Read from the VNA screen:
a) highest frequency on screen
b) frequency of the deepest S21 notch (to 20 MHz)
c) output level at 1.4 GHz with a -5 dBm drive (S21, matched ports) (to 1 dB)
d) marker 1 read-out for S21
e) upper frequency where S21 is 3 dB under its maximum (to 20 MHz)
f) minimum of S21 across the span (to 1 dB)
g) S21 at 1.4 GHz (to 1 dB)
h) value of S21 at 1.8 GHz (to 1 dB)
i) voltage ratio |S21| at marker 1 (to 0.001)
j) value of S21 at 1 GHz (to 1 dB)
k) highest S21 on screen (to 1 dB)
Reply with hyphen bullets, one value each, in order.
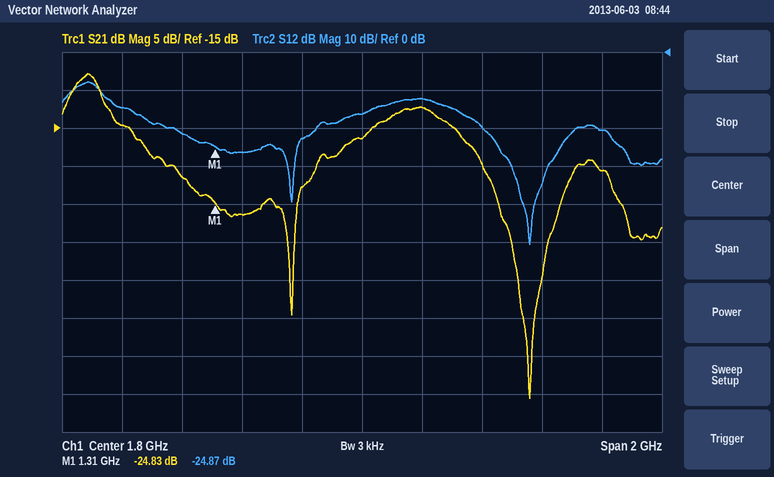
- 2.8 GHz
- 2.36 GHz
- -31 dBm
- -24.83 dB
- 940 MHz
- -51 dB
- -26 dB
- -16 dB
- 0.057
- -15 dB
- -8 dB
